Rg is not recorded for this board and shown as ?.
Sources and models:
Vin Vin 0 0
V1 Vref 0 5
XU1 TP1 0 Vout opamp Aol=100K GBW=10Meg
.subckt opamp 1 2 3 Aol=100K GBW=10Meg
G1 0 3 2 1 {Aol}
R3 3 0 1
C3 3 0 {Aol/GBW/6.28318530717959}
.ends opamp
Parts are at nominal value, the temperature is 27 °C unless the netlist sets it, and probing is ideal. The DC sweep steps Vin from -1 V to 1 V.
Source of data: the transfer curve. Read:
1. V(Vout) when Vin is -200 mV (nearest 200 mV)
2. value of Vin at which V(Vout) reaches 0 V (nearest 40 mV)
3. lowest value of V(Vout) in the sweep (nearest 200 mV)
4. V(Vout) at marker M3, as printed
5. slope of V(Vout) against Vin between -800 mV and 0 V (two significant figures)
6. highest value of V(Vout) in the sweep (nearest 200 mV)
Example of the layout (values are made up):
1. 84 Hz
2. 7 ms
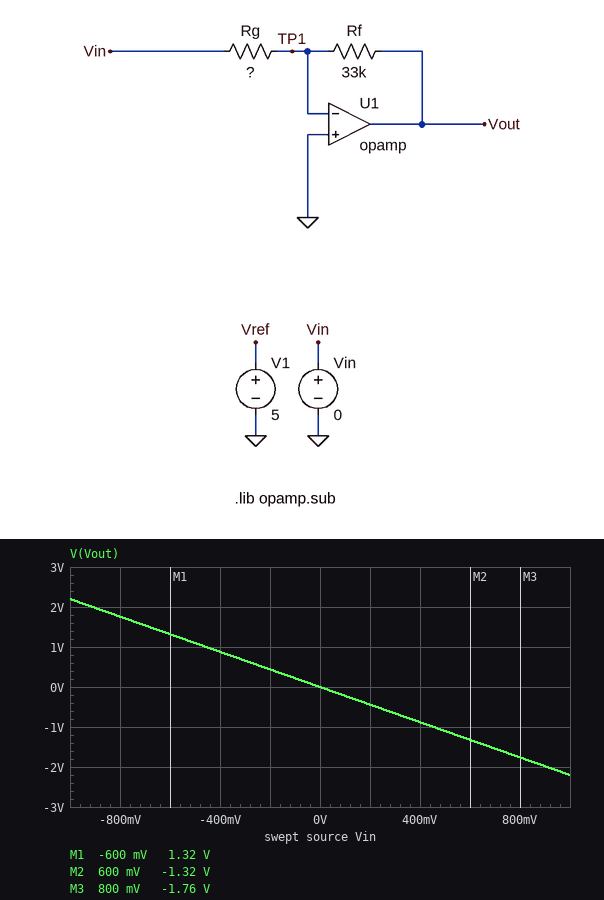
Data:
1. 400 mV
2. 0 V
3. -2.2 V
4. -1.76 V
5. -2.2 V/V
6. 2.2 V
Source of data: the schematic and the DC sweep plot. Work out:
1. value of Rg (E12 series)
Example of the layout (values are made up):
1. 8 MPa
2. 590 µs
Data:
1. 15 kΩ
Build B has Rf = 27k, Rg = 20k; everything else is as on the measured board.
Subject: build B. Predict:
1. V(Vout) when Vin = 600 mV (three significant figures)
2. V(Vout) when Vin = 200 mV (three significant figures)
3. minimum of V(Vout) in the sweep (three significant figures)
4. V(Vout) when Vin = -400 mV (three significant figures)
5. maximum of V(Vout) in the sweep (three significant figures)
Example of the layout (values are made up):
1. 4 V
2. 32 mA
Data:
1. -810 mV
2. -270 mV
3. -1.35 V
4. 540 mV
5. 1.35 V
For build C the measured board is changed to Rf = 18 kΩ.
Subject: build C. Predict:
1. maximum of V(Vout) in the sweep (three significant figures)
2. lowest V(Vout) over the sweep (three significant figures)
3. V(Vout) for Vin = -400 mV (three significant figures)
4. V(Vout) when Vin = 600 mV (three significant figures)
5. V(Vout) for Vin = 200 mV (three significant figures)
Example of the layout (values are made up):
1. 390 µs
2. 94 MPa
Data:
1. 1.20 V
2. -1.20 V
3. 480 mV
4. -720 mV
5. -240 mV
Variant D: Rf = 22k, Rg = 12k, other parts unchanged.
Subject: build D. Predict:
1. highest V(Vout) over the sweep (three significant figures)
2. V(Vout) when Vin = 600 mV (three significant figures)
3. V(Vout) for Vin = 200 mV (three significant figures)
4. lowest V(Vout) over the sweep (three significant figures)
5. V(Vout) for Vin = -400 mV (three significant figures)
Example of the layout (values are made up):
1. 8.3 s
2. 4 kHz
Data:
1. 1.83 V
2. -1.10 V
3. -367 mV
4. -1.83 V
5. 733 mV
